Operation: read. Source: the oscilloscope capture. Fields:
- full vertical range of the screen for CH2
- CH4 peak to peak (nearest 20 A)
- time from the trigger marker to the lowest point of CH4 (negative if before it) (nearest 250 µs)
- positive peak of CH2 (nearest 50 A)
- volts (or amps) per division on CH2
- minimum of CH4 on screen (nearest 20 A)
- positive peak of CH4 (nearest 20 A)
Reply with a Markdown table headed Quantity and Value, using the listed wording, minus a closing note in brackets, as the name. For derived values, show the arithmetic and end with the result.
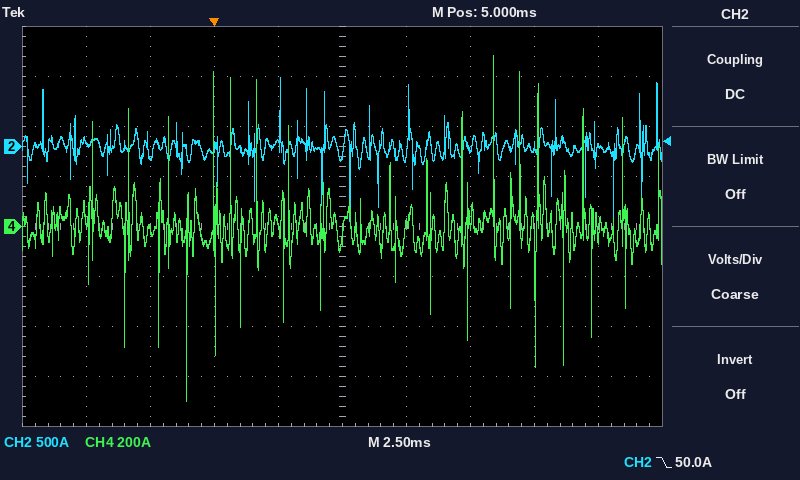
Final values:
| Quantity | Value |
|---|---|
| full vertical range of the screen for CH2 | 4 kA |
| CH4 peak to peak | 680 A − (-700 A) = 1.38 kA |
| time from the trigger marker to the lowest point of CH4 (negative if before it) | -1.00 ms |
| positive peak of CH2 | 700 A |
| volts (or amps) per division on CH2 | 500 A |
| minimum of CH4 on screen | -700 A |
| positive peak of CH4 | 680 A |
